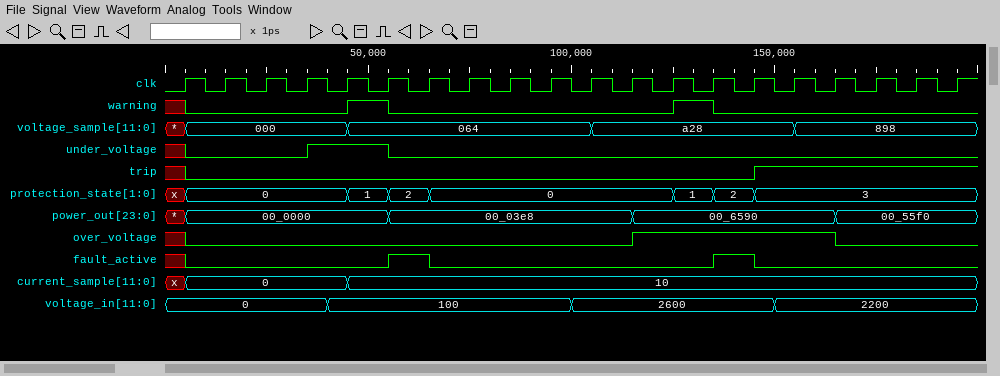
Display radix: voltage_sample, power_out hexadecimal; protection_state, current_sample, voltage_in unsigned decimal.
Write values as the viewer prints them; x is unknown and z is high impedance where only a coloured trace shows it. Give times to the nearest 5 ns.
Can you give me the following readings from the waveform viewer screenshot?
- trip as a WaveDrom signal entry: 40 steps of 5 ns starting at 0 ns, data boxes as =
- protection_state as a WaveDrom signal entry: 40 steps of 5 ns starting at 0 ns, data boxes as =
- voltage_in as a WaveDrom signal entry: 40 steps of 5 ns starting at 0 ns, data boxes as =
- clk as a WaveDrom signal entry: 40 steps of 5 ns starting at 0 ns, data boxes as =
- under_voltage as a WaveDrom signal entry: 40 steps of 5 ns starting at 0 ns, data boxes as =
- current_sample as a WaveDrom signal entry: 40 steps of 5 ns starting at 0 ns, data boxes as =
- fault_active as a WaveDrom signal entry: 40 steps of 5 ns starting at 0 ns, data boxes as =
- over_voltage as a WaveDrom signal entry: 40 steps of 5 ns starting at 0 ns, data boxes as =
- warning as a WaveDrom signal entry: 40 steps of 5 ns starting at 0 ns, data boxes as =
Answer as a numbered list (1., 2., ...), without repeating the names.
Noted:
1. {name: 'trip', wave: 'x0...........................1..........'}
2. {name: 'protection_state', wave: 'x=.......=.=.=...........=.=.=..........', data: '0 1 2 0 1 2 3'}
3. {name: 'voltage_in', wave: '=.......=...........=.........=.........', data: '0 100 2600 2200'}
4. {name: 'clk', wave: '0101010101010101010101010101010101010101'}
5. {name: 'under_voltage', wave: 'x0.....1...0............................'}
6. {name: 'current_sample', wave: 'x=.......=..............................', data: '0 10'}
7. {name: 'fault_active', wave: 'x0.........1.0.............1.0..........'}
8. {name: 'over_voltage', wave: 'x0.....................1.........0......'}
9. {name: 'warning', wave: 'x0.......1.0.............1.0............'}
